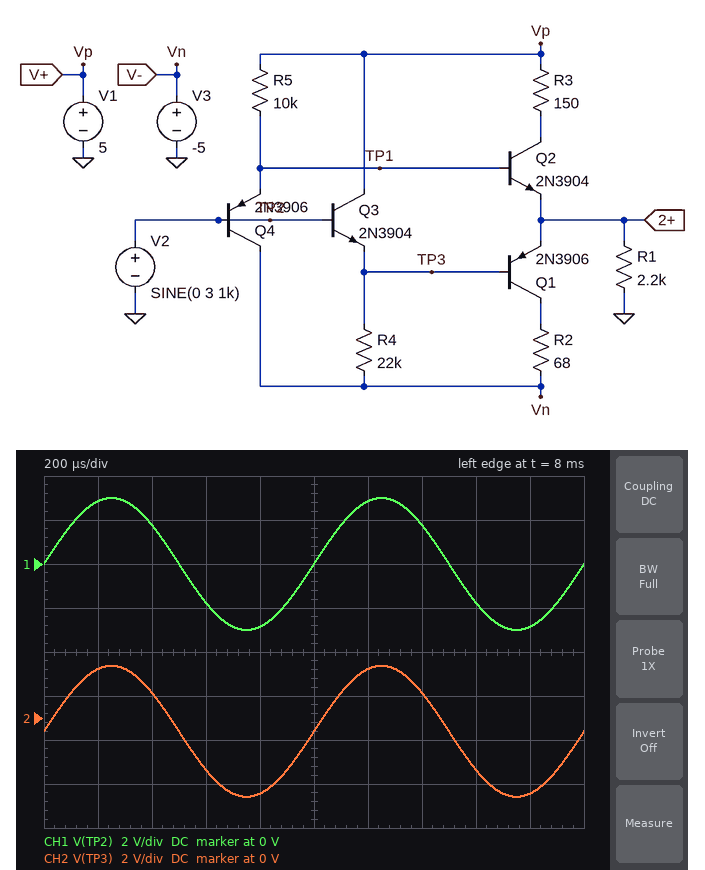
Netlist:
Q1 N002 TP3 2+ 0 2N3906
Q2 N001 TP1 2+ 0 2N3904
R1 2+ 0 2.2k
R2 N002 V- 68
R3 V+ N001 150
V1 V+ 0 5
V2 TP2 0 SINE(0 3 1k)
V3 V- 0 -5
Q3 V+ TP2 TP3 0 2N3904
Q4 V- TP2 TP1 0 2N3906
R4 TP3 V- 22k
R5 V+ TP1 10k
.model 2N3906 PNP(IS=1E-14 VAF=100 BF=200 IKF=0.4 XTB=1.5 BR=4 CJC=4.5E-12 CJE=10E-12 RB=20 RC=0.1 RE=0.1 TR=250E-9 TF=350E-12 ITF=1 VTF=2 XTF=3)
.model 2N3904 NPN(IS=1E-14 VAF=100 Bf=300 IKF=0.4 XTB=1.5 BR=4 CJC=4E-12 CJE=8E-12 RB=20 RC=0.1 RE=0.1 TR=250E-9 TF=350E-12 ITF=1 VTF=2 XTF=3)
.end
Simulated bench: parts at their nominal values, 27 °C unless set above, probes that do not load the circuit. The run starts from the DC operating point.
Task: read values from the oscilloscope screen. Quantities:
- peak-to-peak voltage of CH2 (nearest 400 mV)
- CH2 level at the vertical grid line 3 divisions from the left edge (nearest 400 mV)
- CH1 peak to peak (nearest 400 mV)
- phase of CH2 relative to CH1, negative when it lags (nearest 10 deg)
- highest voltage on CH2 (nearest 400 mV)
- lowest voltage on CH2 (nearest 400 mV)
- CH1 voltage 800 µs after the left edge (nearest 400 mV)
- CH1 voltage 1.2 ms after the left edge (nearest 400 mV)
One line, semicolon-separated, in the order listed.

6.0 V; -2.4 V; 6.0 V; 0 deg; 2.4 V; -3.6 V; -2.8 V; 2.8 V
